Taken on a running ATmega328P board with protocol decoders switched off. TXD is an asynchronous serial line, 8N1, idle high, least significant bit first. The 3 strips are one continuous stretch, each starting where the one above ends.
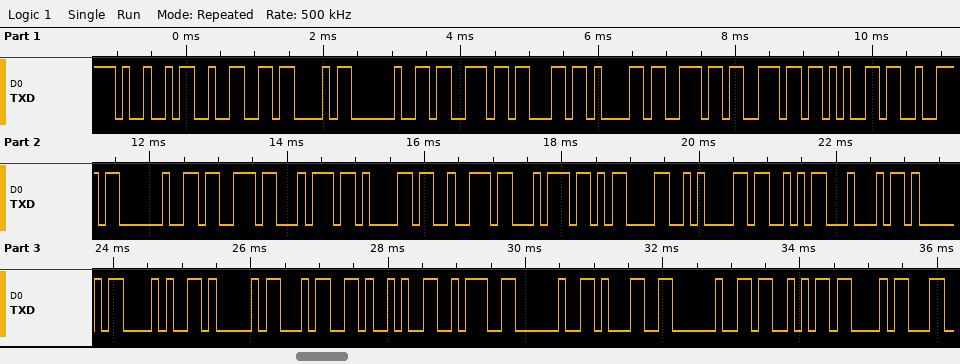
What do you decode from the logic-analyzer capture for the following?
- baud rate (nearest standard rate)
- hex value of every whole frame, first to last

9600 baud
49 32 43 20 73 63 61 6E 6E 65 72 20 73 74 61 72 74 0D 0A 53 44 41 28 41 34 29 3A 20 31 20 53 43
